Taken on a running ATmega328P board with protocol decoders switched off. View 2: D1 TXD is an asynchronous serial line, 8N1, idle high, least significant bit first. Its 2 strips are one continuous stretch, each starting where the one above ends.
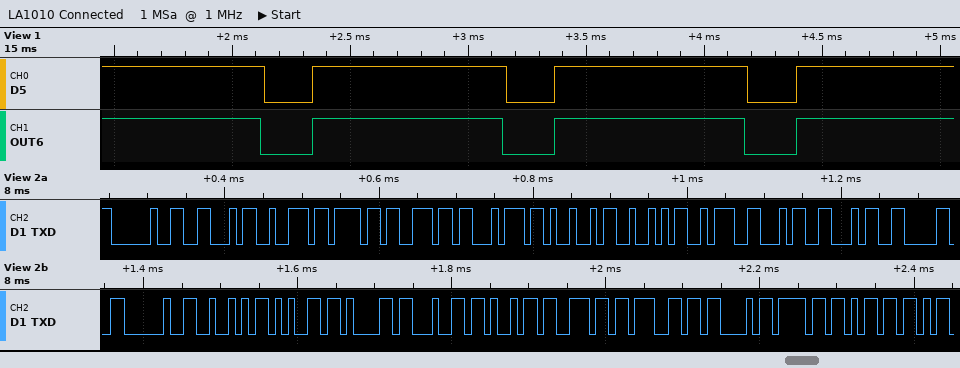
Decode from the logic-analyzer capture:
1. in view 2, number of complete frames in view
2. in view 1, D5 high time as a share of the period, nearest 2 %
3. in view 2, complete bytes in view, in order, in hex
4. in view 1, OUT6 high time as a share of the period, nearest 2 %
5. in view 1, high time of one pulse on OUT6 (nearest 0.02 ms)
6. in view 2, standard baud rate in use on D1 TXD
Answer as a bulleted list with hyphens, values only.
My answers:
- 23
- 80 %
- 20 46 72 6F 6E 74 49 52 3A 34 34 30 20 52 65 61 64 69 6E 67 43 6F 6D
- 78 %
- 0.80 ms
- 115200 baud
